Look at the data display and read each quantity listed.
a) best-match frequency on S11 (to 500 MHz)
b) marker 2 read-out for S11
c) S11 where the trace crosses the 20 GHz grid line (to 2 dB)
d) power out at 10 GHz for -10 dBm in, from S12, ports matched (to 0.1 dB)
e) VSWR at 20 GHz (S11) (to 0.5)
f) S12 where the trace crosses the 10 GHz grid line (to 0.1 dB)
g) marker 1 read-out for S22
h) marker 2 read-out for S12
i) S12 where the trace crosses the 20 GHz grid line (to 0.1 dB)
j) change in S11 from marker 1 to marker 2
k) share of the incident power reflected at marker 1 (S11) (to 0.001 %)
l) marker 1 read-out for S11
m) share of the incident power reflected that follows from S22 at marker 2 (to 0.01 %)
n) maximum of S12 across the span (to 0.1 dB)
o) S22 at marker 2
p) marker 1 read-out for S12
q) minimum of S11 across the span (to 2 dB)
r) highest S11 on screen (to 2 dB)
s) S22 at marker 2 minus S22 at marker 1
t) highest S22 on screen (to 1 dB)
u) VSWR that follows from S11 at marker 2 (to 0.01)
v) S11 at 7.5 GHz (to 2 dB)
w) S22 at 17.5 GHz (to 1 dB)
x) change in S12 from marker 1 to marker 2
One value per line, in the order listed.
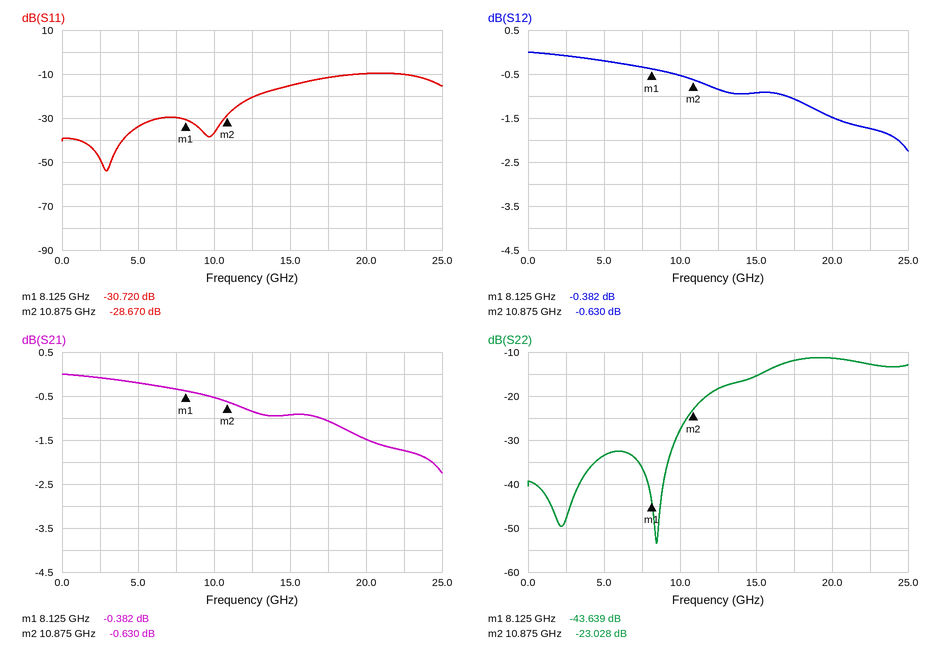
3.0 GHz
-28.670 dB
-10 dB
-10.5 dBm
2.0
-0.5 dB
-43.639 dB
-0.630 dB
-1.5 dB
2.050 dB
0.085 %
-30.720 dB
0.50 %
0.0 dB
-23.028 dB
-0.382 dB
-54 dB
-10 dB
20.611 dB
-11 dB
1.08
-30 dB
-12 dB
-0.248 dB
